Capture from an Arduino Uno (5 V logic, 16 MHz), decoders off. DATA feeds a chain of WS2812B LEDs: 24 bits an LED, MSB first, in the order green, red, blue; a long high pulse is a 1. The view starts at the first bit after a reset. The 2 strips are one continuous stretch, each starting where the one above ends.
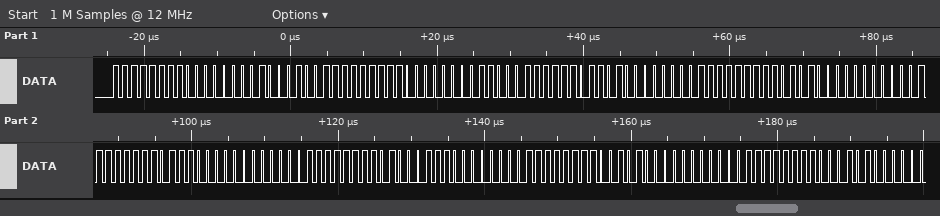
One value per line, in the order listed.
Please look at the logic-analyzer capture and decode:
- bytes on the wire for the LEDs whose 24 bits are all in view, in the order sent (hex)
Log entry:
FF 00 89 FF 00 C7 ED 00 FF A8 00 FF 70 00 FF 47 00 FF 28 00 FF
